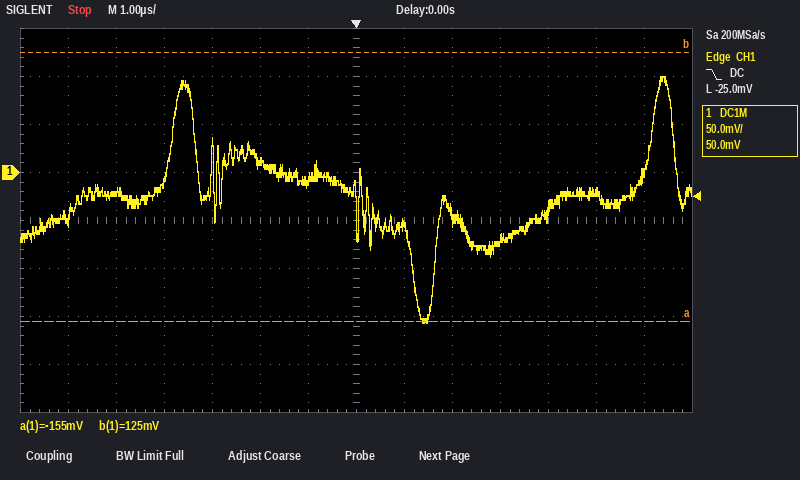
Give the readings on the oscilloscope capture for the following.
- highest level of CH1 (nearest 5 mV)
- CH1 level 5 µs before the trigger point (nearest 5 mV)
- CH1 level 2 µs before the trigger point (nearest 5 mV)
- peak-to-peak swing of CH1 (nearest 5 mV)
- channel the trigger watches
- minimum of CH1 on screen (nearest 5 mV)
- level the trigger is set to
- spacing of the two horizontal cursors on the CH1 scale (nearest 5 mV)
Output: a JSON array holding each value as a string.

["100 mV", "-20 mV", "10 mV", "255 mV", "CH1", "-155 mV", "-25.0 mV", "280 mV"]
